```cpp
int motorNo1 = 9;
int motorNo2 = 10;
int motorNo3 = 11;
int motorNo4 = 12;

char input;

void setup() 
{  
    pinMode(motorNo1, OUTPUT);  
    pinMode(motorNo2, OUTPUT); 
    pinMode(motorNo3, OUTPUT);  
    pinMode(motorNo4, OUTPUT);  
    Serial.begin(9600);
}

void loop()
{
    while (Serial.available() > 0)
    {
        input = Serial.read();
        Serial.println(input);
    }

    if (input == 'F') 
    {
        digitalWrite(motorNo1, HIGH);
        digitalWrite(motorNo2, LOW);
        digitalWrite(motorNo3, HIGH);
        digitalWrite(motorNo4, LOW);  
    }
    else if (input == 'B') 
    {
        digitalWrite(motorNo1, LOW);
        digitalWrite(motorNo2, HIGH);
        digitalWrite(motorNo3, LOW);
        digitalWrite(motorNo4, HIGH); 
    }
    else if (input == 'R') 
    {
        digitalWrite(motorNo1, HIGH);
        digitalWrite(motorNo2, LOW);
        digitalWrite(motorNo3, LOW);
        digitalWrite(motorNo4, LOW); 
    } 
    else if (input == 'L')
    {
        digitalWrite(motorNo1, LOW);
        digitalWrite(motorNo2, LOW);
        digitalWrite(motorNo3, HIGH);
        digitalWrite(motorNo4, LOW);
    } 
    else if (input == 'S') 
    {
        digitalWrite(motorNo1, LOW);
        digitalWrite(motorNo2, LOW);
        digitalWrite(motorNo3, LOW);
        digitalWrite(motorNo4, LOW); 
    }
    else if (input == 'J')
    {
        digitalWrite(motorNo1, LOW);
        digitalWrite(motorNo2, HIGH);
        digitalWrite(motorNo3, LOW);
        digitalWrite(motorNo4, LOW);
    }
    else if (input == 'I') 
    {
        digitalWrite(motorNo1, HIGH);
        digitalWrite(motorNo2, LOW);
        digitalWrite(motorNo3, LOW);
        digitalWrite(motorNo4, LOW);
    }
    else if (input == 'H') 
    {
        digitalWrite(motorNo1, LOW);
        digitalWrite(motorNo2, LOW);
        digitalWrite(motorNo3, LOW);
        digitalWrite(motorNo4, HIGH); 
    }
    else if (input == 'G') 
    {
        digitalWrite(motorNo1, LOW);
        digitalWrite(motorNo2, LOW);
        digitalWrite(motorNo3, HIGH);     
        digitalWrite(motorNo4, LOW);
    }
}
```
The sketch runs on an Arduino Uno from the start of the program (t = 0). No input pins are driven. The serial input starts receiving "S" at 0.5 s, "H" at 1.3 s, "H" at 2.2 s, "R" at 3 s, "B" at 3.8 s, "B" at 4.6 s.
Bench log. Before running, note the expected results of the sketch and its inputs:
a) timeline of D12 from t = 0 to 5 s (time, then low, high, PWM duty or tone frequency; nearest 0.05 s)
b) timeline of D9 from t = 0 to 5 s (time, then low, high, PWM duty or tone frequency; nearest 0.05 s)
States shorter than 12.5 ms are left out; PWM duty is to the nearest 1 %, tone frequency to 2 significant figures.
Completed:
0 s low; 1.3 s high; 3 s low; 3.8 s high
0 s low; 3 s high; 3.8 s low
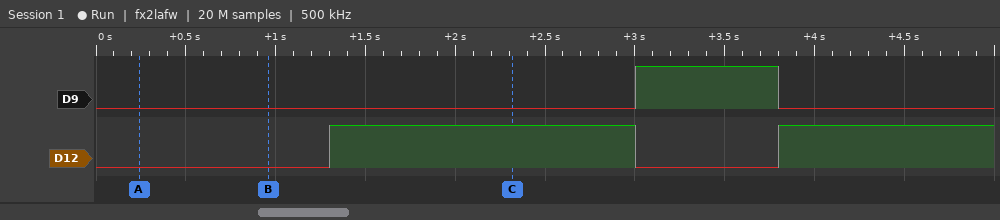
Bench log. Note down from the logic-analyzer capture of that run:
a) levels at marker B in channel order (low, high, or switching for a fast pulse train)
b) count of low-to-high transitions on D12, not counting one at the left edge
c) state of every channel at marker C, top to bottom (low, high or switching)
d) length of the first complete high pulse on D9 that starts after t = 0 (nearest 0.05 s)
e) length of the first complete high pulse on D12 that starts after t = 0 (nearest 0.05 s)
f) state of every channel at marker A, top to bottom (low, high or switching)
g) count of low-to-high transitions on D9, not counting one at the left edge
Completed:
D9 low, D12 low
2
D9 low, D12 high
0.80 s
1.70 s
D9 low, D12 low
1
